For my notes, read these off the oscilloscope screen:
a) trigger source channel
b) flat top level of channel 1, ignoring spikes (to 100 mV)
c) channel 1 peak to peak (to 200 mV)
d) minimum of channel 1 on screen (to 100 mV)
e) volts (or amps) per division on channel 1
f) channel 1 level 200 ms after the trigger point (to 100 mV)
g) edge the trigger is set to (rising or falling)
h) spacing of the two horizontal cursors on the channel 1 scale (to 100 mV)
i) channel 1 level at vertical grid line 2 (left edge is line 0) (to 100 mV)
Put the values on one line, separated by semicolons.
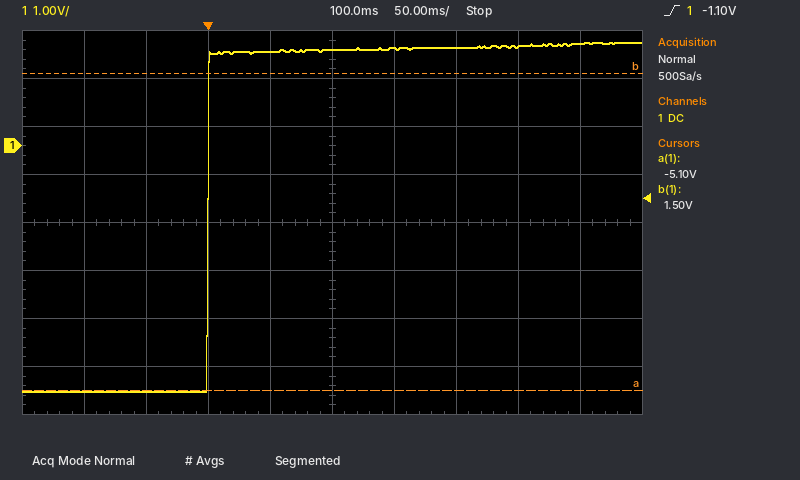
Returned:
channel 1; 2.0 V; 7.2 V; -5.1 V; 1 V; 2.0 V; rising; 6.6 V; -5.1 V
